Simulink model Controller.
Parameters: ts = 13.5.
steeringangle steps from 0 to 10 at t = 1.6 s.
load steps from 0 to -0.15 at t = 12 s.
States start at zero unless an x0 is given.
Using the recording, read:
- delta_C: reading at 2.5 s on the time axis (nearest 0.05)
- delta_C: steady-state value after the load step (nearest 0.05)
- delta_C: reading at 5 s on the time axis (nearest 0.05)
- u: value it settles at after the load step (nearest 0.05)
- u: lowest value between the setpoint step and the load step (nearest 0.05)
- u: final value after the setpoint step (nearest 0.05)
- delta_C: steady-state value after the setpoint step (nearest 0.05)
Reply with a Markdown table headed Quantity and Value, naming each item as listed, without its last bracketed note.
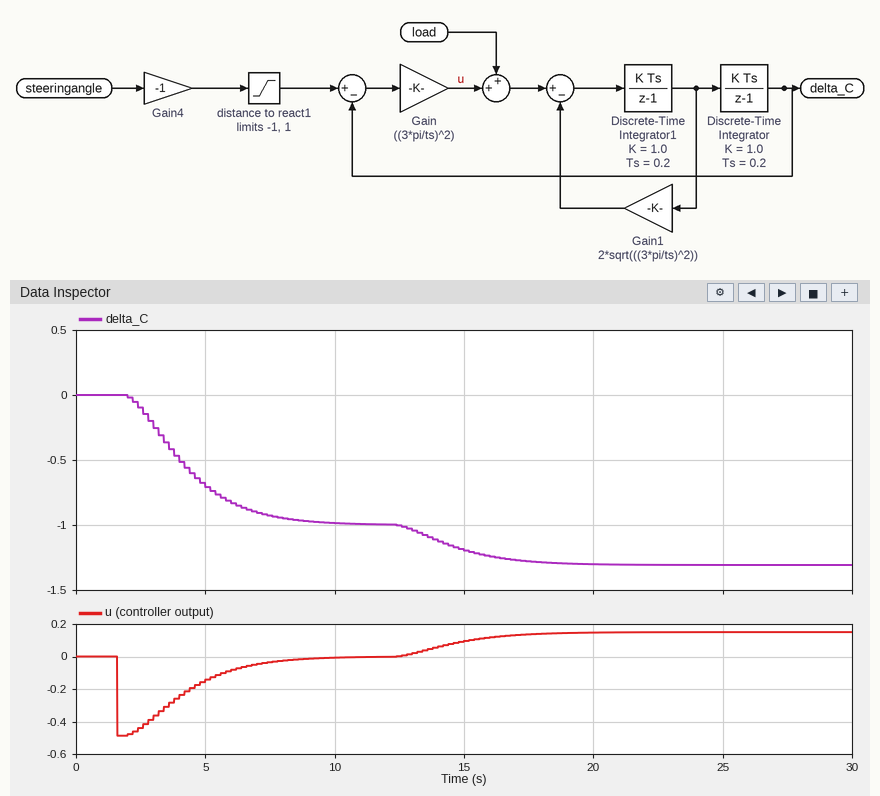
| Quantity | Value |
|---|---|
| delta_C: reading at 2.5 s on the time axis | -0.10 |
| delta_C: steady-state value after the load step | -1.30 |
| delta_C: reading at 5 s on the time axis | -0.70 |
| u: value it settles at after the load step | 0.15 |
| u: lowest value between the setpoint step and the load step | -0.50 |
| u: final value after the setpoint step | 0.00 |
| delta_C: steady-state value after the setpoint step | -1.00 |
